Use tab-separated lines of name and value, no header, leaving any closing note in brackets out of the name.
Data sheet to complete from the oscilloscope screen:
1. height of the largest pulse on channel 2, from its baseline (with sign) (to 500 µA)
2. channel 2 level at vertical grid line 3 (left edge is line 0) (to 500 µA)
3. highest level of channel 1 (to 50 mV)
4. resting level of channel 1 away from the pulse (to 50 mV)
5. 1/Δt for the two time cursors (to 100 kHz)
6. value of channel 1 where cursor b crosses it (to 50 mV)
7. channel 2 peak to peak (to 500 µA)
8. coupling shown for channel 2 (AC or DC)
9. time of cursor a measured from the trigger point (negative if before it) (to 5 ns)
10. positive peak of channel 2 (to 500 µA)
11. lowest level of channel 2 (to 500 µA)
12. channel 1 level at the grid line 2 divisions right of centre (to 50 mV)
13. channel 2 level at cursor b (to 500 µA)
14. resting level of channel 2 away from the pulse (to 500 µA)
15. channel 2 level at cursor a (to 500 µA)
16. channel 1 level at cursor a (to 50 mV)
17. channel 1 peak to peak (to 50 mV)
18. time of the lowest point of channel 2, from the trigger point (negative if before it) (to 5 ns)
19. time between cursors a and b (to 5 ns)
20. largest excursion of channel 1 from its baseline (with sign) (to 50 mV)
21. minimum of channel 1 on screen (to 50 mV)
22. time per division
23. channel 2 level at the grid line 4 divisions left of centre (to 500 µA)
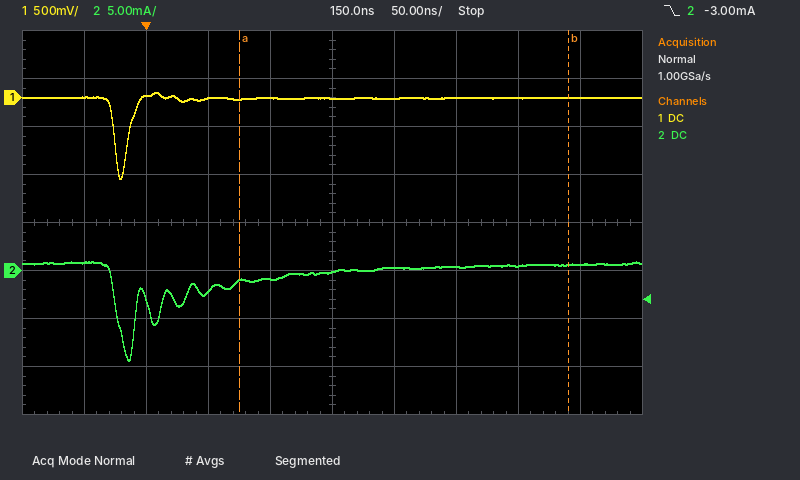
height of the largest pulse on channel 2, from its baseline (with sign)	-10.0 mA
channel 2 level at vertical grid line 3 (left edge is line 0)	-2.0 mA
highest level of channel 1	50 mV
resting level of channel 1 away from the pulse	0 mV
1/Δt for the two time cursors	3.8 MHz
value of channel 1 where cursor b crosses it	0 mV
channel 2 peak to peak	10.5 mA
coupling shown for channel 2	DC
time of cursor a measured from the trigger point (negative if before it)	+75 ns
positive peak of channel 2	1.0 mA
lowest level of channel 2	-9.5 mA
channel 1 level at the grid line 2 divisions right of centre	0 mV
channel 2 level at cursor b	500 µA
resting level of channel 2 away from the pulse	500 µA
channel 2 level at cursor a	-1.0 mA
channel 1 level at cursor a	0 mV
channel 1 peak to peak	900 mV
time of the lowest point of channel 2, from the trigger point (negative if before it)	-15 ns
time between cursors a and b	265 ns
largest excursion of channel 1 from its baseline (with sign)	-850 mV
minimum of channel 1 on screen	-850 mV
time per division	50 ns
channel 2 level at the grid line 4 divisions left of centre	1.0 mA
